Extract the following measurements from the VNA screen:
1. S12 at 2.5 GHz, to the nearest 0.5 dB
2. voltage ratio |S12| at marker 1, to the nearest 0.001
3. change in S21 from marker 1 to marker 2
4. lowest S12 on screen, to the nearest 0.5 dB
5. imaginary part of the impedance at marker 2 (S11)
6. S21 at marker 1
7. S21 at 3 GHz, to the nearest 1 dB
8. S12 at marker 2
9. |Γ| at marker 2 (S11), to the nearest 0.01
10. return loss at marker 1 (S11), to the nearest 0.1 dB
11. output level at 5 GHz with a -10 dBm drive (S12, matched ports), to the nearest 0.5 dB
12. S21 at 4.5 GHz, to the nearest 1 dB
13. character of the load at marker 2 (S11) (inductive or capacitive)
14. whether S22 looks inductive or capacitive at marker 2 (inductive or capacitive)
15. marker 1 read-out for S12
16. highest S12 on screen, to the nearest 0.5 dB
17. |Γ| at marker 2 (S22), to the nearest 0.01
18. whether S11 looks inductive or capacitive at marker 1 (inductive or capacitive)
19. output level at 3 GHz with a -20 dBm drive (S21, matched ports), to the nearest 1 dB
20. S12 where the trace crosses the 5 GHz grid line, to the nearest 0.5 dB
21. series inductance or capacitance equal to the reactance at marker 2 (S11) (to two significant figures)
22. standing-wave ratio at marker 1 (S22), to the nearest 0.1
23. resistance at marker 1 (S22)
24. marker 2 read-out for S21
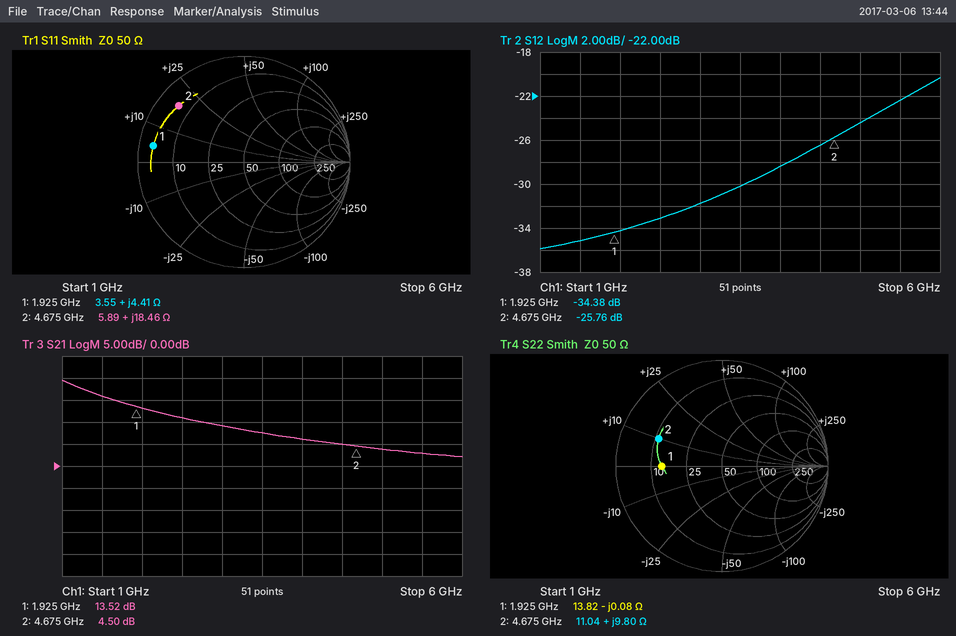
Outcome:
-33.0 dB
0.019
-9.02 dB
-36.0 dB
+18.46 Ω
13.52 dB
9 dB
-25.76 dB
0.81
1.2 dB
-34.5 dBm
5 dB
inductive
inductive
-34.38 dB
-20.5 dB
0.65
inductive
-11 dBm
-24.5 dB
630 pH
3.6
13.82 Ω
4.50 dB
